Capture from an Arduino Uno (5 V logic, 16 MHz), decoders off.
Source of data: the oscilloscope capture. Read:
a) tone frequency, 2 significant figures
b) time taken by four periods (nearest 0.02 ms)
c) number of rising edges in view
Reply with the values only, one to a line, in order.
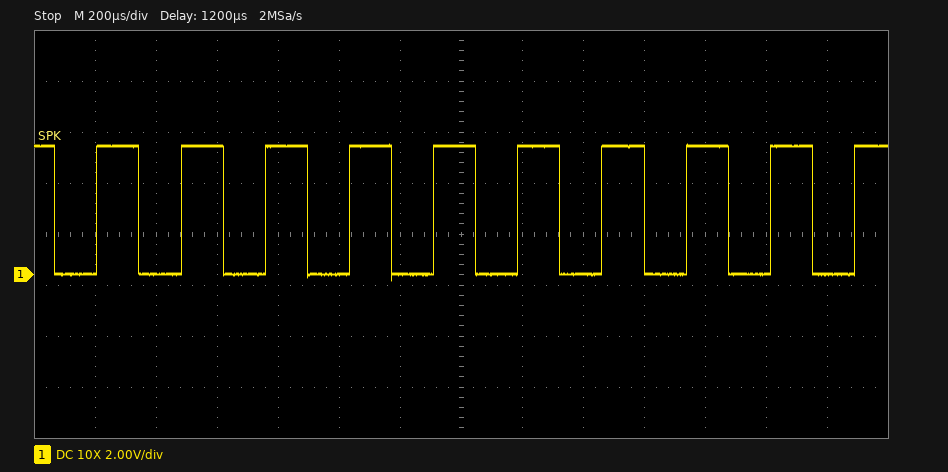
3.6 kHz
1.10 ms
10
